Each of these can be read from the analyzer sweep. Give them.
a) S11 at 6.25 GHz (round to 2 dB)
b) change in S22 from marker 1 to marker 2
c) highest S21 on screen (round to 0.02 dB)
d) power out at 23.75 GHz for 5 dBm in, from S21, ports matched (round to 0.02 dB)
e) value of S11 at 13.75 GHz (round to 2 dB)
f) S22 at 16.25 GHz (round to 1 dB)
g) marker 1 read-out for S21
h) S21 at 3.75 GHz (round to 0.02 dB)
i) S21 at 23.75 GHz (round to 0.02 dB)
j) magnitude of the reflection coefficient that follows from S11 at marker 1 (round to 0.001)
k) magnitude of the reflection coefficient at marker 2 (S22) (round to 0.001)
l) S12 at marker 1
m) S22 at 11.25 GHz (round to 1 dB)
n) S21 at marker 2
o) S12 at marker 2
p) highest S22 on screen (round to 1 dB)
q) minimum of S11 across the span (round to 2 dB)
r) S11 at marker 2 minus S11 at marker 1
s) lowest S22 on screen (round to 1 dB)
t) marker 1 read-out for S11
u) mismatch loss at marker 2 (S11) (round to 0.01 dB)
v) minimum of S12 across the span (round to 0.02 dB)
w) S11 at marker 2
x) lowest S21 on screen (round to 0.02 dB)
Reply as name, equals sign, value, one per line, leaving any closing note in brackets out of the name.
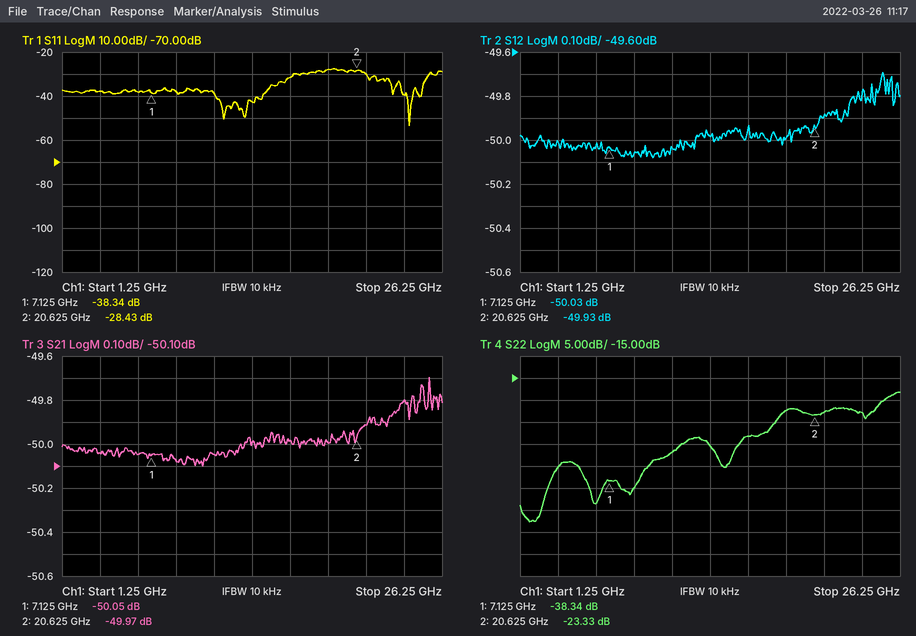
S11 at 6.25 GHz = -38 dB
change in S22 from marker 1 to marker 2 = 15.01 dB
highest S21 on screen = -49.70 dB
power out at 23.75 GHz for 5 dBm in, from S21, ports matched = -44.80 dBm
value of S11 at 13.75 GHz = -42 dB
S22 at 16.25 GHz = -28 dB
marker 1 read-out for S21 = -50.05 dB
S21 at 3.75 GHz = -50.04 dB
S21 at 23.75 GHz = -49.80 dB
magnitude of the reflection coefficient that follows from S11 at marker 1 = 0.012
magnitude of the reflection coefficient at marker 2 (S22) = 0.068
S12 at marker 1 = -50.03 dB
S22 at 11.25 GHz = -32 dB
S21 at marker 2 = -49.97 dB
S12 at marker 2 = -49.93 dB
highest S22 on screen = -18 dB
minimum of S11 across the span = -54 dB
S11 at marker 2 minus S11 at marker 1 = 9.91 dB
lowest S22 on screen = -48 dB
marker 1 read-out for S11 = -38.34 dB
mismatch loss at marker 2 (S11) = 0.01 dB
minimum of S12 across the span = -50.08 dB
S11 at marker 2 = -28.43 dB
lowest S21 on screen = -50.10 dB
